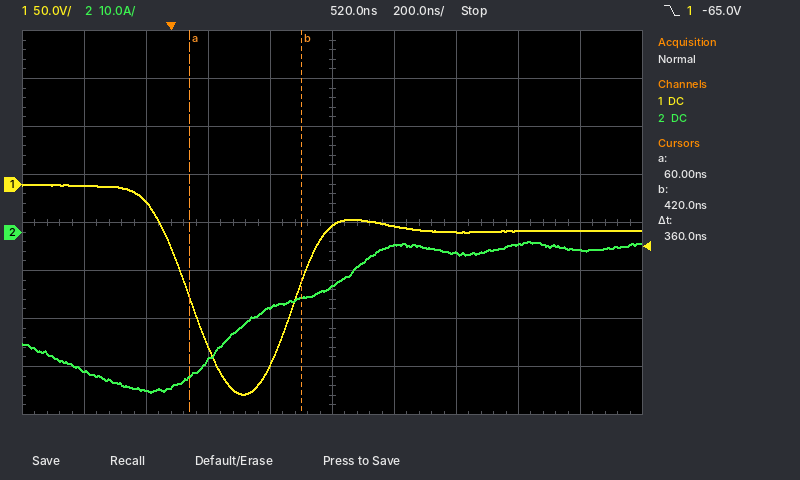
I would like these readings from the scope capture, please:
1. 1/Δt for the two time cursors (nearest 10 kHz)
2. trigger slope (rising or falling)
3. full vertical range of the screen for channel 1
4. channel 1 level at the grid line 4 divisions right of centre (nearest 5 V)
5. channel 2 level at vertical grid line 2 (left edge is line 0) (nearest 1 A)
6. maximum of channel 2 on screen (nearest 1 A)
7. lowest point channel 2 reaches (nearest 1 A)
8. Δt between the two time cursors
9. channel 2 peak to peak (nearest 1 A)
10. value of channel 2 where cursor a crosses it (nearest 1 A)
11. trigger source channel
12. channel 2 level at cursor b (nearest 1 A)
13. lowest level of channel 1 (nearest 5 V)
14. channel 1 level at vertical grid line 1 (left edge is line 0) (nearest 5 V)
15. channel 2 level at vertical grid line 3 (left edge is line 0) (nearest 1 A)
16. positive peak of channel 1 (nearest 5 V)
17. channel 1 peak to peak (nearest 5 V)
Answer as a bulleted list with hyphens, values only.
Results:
- 2.78 MHz
- falling
- 400 V
- -50 V
- -33 A
- -2 A
- -33 A
- 360 ns
- 31 A
- -30 A
- channel 1
- -14 A
- -220 V
- 0 V
- -27 A
- 0 V
- 220 V
